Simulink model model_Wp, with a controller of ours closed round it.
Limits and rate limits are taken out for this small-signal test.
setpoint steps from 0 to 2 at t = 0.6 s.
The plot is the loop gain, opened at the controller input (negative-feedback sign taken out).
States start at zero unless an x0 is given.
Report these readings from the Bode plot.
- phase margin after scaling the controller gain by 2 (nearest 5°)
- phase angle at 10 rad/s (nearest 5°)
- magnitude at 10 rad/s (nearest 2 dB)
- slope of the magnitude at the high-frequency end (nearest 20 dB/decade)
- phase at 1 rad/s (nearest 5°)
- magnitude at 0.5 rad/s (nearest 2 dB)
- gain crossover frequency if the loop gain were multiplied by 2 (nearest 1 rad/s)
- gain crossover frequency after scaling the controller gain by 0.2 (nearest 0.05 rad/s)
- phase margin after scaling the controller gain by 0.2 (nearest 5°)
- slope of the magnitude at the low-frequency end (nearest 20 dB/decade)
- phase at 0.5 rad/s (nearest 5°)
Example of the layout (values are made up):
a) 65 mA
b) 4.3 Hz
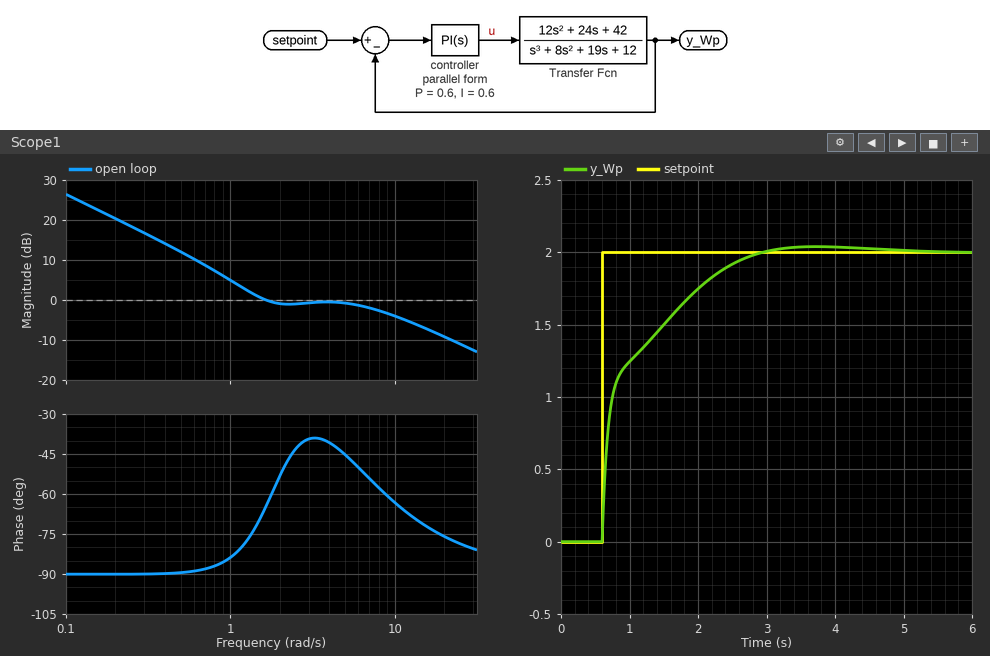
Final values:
a) 110°
b) -65°
c) -4 dB
d) -20 dB/decade
e) -85°
f) 12 dB
g) 13 rad/s
h) 0.40 rad/s
i) 90°
j) -20 dB/decade
k) -90°
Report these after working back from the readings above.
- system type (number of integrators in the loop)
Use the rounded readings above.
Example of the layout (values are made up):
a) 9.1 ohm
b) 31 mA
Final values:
a) 1
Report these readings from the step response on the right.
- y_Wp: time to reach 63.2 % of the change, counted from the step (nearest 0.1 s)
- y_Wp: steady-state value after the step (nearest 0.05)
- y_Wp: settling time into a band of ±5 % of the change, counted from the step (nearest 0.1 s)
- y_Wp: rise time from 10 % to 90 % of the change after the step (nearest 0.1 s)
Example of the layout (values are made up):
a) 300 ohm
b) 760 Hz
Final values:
a) 0.4 s
b) 2.00
c) 1.8 s
d) 1.5 s
